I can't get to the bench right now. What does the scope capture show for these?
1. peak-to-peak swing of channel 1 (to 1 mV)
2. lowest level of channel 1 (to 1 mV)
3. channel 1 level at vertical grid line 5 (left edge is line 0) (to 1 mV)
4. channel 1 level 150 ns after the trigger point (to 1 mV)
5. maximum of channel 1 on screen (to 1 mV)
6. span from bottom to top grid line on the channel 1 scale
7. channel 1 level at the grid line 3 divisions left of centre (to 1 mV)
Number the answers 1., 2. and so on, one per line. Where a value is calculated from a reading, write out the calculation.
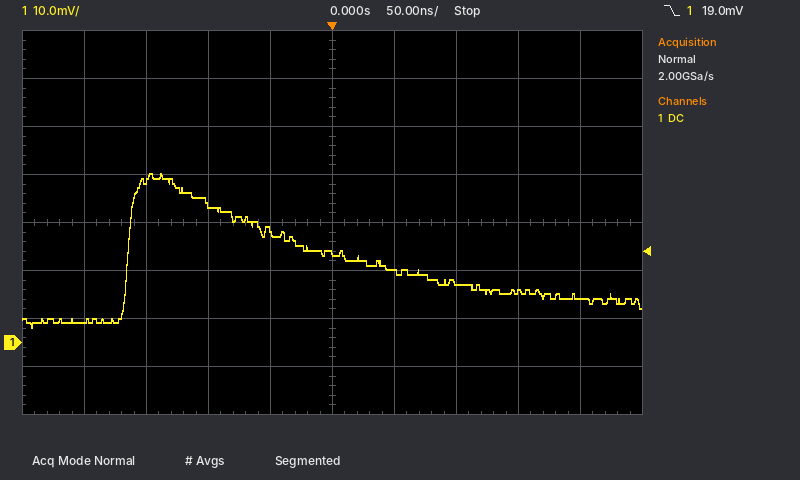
1. 35 mV − (3 mV) = 32 mV
2. 3 mV
3. 19 mV
4. 11 mV
5. 35 mV
6. 80 mV
7. 34 mV
